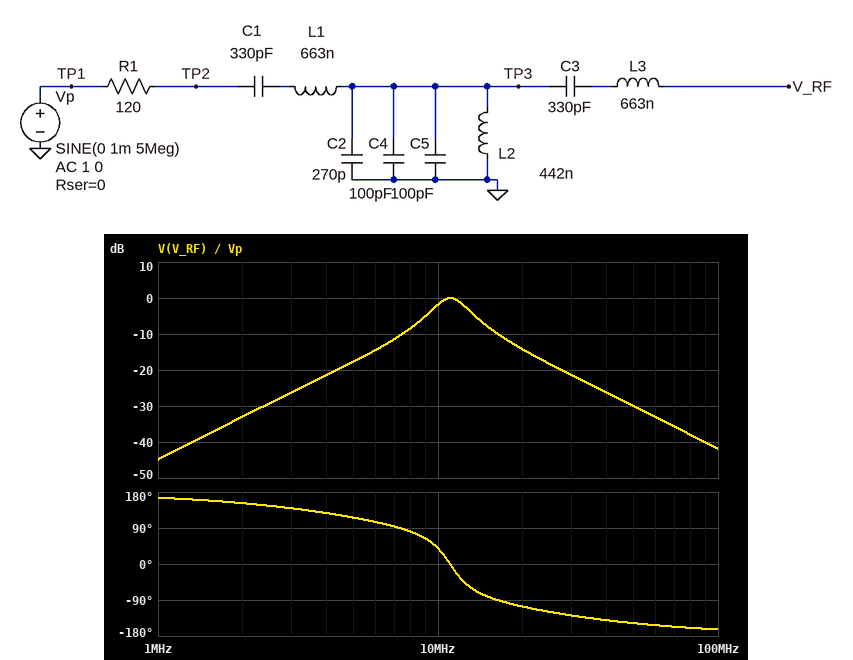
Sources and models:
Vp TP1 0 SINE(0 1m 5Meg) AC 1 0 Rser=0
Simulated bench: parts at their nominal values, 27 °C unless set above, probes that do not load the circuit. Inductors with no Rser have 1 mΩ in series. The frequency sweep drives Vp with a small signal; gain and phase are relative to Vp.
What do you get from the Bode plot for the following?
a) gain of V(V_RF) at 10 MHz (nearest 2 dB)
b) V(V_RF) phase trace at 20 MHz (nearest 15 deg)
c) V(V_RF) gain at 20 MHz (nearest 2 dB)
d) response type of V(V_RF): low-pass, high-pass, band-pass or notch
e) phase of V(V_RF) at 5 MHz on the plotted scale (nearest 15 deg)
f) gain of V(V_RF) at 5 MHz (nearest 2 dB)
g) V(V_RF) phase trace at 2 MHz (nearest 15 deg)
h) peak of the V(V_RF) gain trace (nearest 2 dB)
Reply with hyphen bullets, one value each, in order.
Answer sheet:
- -2 dB
- -105 deg
- -14 dB
- band-pass
- 120 deg
- -18 dB
- 150 deg
- 0 dB
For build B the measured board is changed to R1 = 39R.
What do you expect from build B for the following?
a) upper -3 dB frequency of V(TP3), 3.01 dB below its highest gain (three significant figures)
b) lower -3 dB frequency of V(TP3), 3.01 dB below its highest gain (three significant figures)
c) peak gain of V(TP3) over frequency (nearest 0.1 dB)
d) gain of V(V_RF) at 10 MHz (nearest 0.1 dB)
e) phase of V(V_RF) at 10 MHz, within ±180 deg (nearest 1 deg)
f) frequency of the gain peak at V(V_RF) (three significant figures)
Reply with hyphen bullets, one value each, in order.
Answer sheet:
- 17.3 MHz
- 6.99 MHz
- 1.2 dB
- 0.1 dB
- 15 deg
- 14.4 MHz
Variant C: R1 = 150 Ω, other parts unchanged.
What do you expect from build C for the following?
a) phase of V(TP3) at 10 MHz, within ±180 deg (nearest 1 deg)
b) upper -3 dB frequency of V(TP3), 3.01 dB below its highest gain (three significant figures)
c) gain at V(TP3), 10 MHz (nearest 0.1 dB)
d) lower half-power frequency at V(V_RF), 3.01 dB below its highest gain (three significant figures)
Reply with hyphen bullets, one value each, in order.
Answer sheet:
- 45 deg
- 12.3 MHz
- -2.7 dB
- 9.92 MHz
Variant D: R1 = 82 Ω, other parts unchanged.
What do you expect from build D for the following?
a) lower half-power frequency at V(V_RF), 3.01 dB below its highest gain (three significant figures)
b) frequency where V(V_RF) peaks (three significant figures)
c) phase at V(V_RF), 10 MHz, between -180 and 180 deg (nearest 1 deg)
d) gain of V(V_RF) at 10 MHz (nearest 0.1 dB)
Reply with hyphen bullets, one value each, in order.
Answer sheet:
- 8.83 MHz
- 11.1 MHz
- 29 deg
- -0.8 dB
